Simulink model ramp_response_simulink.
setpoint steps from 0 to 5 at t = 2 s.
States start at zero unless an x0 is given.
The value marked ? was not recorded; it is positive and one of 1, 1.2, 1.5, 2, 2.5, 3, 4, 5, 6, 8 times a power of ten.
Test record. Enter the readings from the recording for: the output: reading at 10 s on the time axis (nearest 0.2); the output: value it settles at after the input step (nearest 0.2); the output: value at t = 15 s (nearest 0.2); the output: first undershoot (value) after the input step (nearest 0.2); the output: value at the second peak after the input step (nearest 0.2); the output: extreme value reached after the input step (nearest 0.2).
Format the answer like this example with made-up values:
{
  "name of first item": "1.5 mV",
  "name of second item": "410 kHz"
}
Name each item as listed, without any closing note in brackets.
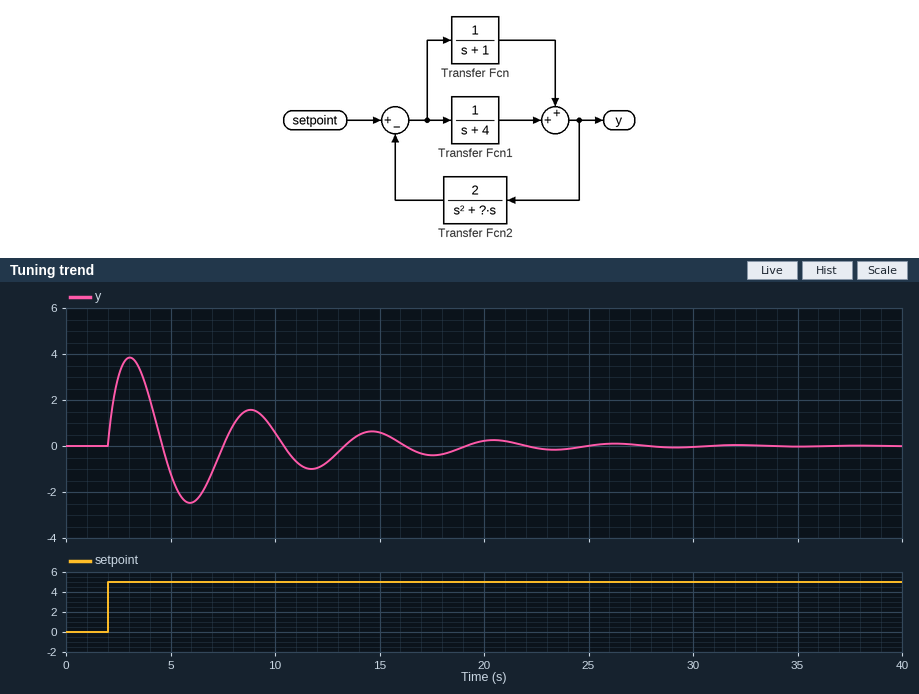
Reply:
{
  "the output: reading at 10 s on the time axis": "0.6",
  "the output: value it settles at after the input step": "0.0",
  "the output: value at t = 15 s": "0.6",
  "the output: first undershoot (value) after the input step": "-2.4",
  "the output: value at the second peak after the input step": "1.6",
  "the output: extreme value reached after the input step": "3.8"
}
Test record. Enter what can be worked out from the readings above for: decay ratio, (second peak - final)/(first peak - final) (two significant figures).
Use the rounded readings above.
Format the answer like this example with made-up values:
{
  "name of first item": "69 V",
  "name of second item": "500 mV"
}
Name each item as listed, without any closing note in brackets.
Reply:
{
  "decay ratio, (second peak - final)/(first peak - final)": "0.42"
}
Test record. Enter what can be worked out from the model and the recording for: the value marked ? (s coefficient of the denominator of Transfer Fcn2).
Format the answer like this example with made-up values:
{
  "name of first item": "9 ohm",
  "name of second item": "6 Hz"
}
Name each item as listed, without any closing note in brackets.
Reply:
{
  "the value marked ?": "1.5"
}
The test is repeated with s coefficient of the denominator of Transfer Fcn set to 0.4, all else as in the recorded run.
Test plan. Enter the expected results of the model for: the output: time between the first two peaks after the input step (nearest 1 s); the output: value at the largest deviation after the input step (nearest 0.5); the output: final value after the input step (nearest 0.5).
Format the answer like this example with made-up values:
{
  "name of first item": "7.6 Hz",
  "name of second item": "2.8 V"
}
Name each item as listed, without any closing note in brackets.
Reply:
{
  "the output: time between the first two peaks after the input step": "5 s",
  "the output: value at the largest deviation after the input step": "5.0",
  "the output: final value after the input step": "0.0"
}
